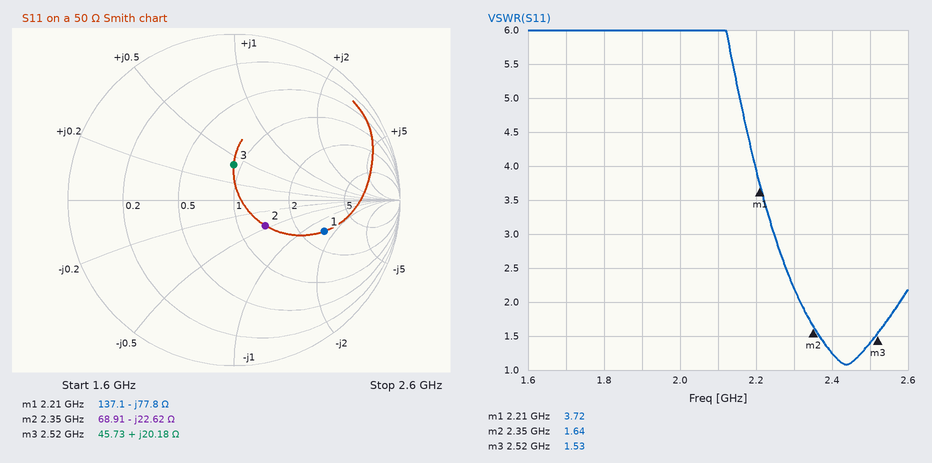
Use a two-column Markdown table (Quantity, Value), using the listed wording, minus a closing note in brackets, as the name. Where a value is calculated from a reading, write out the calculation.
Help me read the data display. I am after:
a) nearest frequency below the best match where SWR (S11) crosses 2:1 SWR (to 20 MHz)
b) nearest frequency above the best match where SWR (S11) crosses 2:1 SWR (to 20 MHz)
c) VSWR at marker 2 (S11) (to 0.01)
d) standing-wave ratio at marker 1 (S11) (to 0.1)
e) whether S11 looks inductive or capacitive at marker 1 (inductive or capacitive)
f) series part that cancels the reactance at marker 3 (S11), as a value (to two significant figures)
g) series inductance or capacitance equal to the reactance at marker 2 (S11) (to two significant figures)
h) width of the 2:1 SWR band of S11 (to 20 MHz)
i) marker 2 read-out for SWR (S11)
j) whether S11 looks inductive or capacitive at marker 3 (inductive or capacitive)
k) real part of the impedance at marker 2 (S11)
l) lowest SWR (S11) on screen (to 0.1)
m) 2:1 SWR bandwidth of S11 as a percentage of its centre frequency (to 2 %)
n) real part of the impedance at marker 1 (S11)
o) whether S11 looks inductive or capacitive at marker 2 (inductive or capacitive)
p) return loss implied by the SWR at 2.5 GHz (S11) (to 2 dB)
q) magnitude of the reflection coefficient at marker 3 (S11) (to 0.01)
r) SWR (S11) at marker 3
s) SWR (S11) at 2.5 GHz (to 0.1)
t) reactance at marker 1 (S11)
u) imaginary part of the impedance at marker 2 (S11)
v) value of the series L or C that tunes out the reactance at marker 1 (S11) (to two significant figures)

| Quantity | Value |
|---|---|
| nearest frequency below the best match where SWR (S11) crosses 2:1 SWR | 2.32 GHz |
| nearest frequency above the best match where SWR (S11) crosses 2:1 SWR | 2.58 GHz |
| VSWR at marker 2 (S11) | 1.64 |
| standing-wave ratio at marker 1 (S11) | 3.7 |
| whether S11 looks inductive or capacitive at marker 1 | capacitive |
| series part that cancels the reactance at marker 3 (S11), as a value | C = 1/(2π × 2.52 GHz × 20.18 Ω) ≈ 3.1 pF |
| series inductance or capacitance equal to the reactance at marker 2 (S11) | C = 1/(2π × 2.35 GHz × 22.62 Ω) ≈ 3.0 pF |
| width of the 2:1 SWR band of S11 | 2.58 GHz − 2.32 GHz = 260 MHz |
| marker 2 read-out for SWR | 1.64 |
| whether S11 looks inductive or capacitive at marker 3 | inductive |
| real part of the impedance at marker 2 | 68.91 Ω |
| lowest SWR (S11) on screen | 1.1 |
| 2:1 SWR bandwidth of S11 as a percentage of its centre frequency | 260 MHz / 2.45 GHz ≈ 10.6 %, so 10 % to the nearest 2 % |
| real part of the impedance at marker 1 | 137.1 Ω |
| whether S11 looks inductive or capacitive at marker 2 | capacitive |
| return loss implied by the SWR at 2.5 GHz (S11) | −20 log10((1.4 − 1)/(1.4 + 1)) ≈ 16 dB |
| magnitude of the reflection coefficient at marker 3 (S11) | 0.21 |
| SWR (S11) at marker 3 | 1.53 |
| SWR (S11) at 2.5 GHz | 1.4 |
| reactance at marker 1 | -77.8 Ω |
| imaginary part of the impedance at marker 2 | -22.62 Ω |
| value of the series L or C that tunes out the reactance at marker 1 (S11) | L = 77.8 Ω/(2π × 2.21 GHz) ≈ 5.6 nH |
